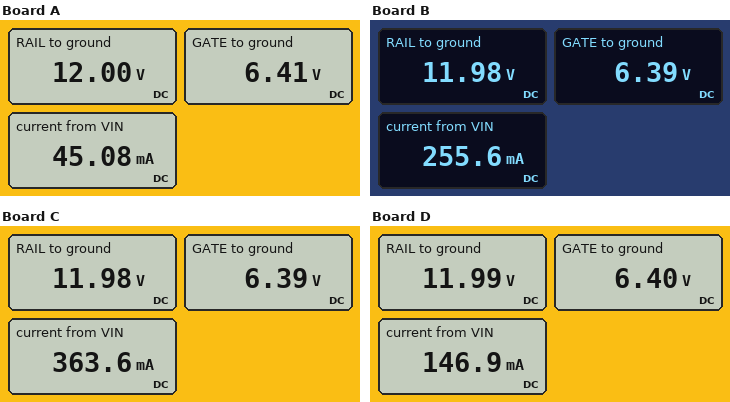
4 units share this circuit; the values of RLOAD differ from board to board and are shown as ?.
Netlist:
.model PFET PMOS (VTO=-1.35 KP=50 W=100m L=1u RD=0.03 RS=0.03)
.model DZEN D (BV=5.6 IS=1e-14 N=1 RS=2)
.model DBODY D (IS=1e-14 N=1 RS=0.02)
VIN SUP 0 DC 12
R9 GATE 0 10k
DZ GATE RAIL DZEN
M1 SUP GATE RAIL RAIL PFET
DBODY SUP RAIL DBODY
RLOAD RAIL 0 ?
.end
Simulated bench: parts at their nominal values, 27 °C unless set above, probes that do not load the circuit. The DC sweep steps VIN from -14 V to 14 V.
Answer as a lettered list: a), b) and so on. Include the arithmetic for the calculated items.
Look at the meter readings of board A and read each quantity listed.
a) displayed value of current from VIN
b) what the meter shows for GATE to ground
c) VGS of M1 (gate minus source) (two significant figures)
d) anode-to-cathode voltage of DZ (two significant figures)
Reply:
a) 45.08 mA
b) 6.41 V
c) 6.41 V - 12 V = -5.6 V
d) 6.41 V - 12 V = -5.6 V
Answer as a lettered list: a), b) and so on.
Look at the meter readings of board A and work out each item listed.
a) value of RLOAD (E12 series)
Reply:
a) 270 Ω
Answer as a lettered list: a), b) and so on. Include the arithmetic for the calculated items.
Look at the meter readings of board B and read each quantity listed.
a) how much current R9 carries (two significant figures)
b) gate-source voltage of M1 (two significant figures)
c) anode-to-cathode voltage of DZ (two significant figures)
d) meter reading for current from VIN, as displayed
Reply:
a) (6.39 V) / 10 kΩ = 640 µA
b) 6.39 V - 11.98 V = -5.6 V
c) 6.39 V - 11.98 V = -5.6 V
d) 255.6 mA
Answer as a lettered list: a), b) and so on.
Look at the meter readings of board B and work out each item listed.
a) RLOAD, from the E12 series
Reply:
a) 47 Ω
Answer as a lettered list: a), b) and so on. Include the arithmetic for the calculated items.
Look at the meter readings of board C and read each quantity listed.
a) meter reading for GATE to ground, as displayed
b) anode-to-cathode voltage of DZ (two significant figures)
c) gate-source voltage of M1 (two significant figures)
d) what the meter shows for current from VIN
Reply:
a) 6.39 V
b) 6.39 V - 11.98 V = -5.6 V
c) 6.39 V - 11.98 V = -5.6 V
d) 363.6 mA
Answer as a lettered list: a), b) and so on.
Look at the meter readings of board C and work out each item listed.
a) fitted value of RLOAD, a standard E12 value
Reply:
a) 33 Ω
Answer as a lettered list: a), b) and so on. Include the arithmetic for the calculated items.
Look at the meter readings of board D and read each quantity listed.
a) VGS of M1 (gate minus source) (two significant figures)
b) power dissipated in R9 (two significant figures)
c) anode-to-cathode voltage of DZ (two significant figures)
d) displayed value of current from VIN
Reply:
a) 6.4 V - 11.99 V = -5.6 V
b) (6.4 V)^2 / 10 kΩ = 4.1 mW
c) 6.4 V - 11.99 V = -5.6 V
d) 146.9 mA
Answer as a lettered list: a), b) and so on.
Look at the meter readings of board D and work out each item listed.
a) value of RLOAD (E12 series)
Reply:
a) 82 Ω
